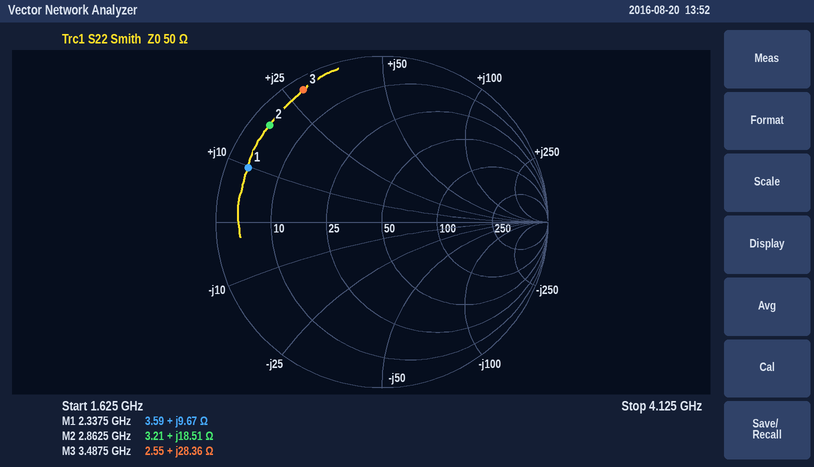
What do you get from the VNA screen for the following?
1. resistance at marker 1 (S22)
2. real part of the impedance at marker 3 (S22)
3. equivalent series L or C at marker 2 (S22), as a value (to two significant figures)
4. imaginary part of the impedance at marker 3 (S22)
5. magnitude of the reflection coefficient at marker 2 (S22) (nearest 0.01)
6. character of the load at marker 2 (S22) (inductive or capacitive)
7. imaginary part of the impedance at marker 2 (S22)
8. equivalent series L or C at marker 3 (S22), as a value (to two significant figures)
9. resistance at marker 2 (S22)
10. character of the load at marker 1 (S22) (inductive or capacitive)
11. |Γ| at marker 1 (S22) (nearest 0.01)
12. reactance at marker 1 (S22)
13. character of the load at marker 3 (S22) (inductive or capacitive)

3.59 Ω
2.55 Ω
1.0 nH
+28.36 Ω
0.89
inductive
+18.51 Ω
1.3 nH
3.21 Ω
inductive
0.87
+9.67 Ω
inductive
